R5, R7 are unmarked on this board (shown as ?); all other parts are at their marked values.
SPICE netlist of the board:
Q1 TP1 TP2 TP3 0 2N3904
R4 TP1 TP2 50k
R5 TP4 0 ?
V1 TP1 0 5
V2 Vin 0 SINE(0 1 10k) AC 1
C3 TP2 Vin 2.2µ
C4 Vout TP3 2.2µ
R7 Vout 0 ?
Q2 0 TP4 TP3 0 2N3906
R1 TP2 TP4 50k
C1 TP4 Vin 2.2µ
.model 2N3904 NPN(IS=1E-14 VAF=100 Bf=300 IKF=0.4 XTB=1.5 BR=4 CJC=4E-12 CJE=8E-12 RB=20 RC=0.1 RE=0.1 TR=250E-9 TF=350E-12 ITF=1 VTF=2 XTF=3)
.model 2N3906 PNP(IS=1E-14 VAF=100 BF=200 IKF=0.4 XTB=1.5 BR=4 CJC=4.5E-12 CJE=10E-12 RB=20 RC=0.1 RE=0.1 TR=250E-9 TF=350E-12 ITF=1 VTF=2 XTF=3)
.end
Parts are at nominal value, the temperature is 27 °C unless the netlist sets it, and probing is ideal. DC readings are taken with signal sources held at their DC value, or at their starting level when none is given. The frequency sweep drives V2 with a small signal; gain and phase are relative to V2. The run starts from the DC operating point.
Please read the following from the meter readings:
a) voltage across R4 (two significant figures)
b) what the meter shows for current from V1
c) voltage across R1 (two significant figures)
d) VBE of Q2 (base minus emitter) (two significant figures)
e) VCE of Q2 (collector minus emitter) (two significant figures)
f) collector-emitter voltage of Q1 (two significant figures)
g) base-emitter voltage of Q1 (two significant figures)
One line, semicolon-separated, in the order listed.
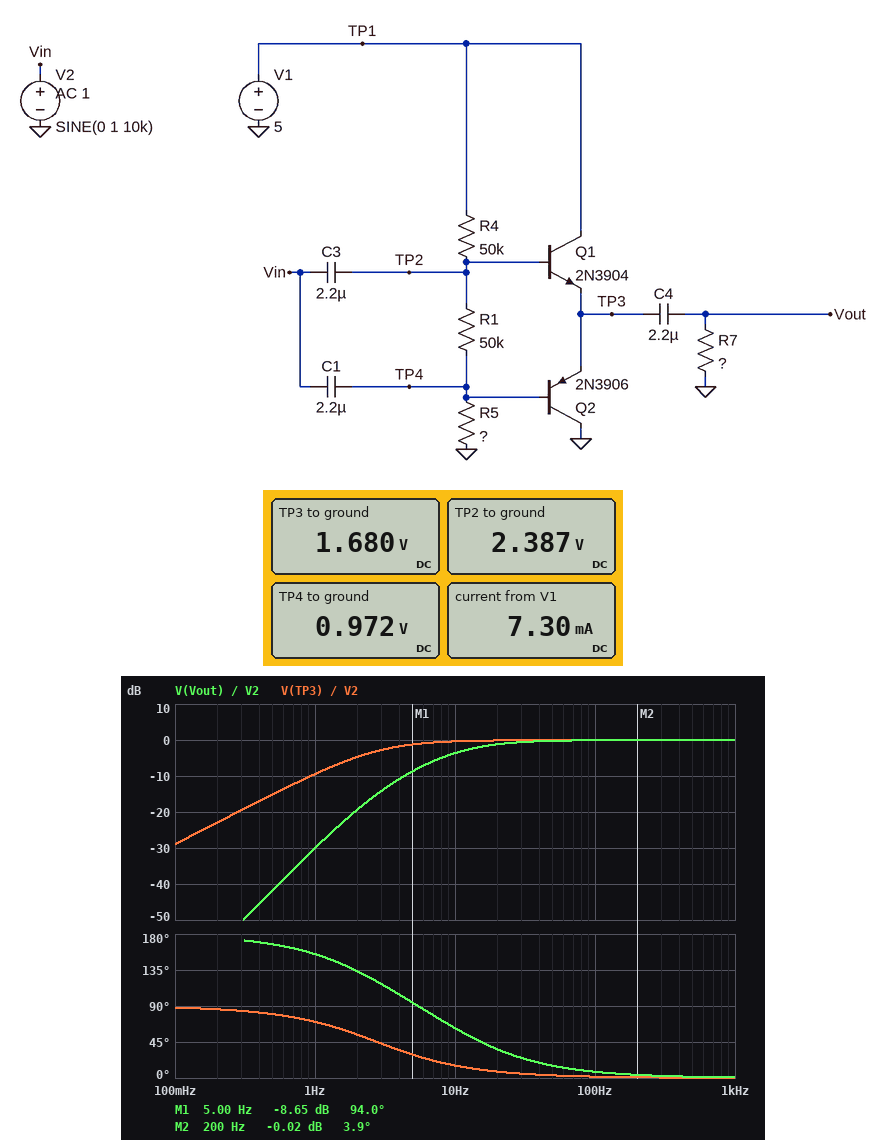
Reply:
2.6 V; 7.30 mA; 1.4 V; -710 mV; -1.7 V; 3.3 V; 710 mV
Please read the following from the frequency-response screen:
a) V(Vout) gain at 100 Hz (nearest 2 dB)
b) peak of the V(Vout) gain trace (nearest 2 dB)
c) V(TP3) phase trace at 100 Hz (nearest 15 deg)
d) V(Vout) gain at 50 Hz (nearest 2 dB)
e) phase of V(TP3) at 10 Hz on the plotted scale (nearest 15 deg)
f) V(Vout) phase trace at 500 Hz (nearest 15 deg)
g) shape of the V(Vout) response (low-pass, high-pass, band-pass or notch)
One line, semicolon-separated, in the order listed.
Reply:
0 dB; 0 dB; 0 deg; 0 dB; 15 deg; 0 deg; high-pass
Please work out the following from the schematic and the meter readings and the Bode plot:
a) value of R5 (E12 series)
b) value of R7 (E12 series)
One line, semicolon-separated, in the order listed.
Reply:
15 kΩ; 6.8 kΩ
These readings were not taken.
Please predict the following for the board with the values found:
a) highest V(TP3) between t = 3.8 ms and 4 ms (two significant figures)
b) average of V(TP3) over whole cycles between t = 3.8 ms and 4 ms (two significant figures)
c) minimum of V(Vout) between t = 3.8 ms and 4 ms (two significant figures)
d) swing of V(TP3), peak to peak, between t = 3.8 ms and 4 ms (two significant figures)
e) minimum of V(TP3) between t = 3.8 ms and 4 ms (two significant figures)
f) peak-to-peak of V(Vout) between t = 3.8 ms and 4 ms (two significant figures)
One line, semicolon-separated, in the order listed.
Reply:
2.7 V; 1.7 V; -1.0 V; 2.0 V; 680 mV; 2.0 V
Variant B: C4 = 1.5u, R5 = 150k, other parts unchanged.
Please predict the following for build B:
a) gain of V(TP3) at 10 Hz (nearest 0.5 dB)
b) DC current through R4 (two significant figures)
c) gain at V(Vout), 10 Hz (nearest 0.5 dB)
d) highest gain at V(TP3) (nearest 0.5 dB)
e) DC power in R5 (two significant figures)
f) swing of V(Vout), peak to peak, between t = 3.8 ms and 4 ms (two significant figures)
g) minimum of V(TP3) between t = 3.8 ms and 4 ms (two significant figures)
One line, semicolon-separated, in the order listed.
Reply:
-2.0 dB; 20 µA; -7.5 dB; -1.0 dB; 60 µW; 1.8 V; 2.6 V
